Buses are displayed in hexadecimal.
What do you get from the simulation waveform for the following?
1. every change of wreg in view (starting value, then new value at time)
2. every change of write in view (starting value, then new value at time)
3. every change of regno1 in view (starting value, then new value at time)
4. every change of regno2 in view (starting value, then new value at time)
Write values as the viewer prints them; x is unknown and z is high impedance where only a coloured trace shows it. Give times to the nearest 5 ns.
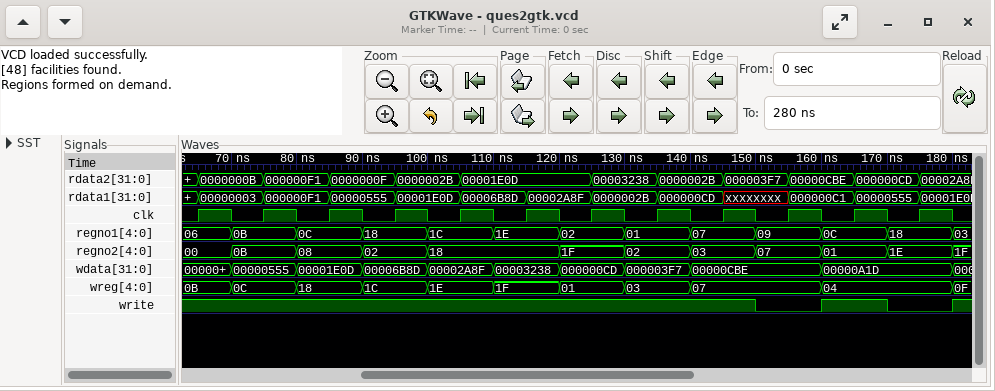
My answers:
0B, 0C at 70 ns, 18 at 80 ns, 1C at 90 ns, 1E at 100 ns, 1F at 110 ns, 01 at 120 ns, 03 at 130 ns, 07 at 140 ns, 04 at 160 ns, 0F at 180 ns
1, 0 at 150 ns, 1 at 160 ns, 0 at 170 ns, 1 at 180 ns
06, 0B at 70 ns, 0C at 80 ns, 18 at 90 ns, 1C at 100 ns, 1E at 110 ns, 02 at 120 ns, 01 at 130 ns, 07 at 140 ns, 09 at 150 ns, 0C at 160 ns, 18 at 170 ns, 03 at 180 ns
00, 0B at 70 ns, 08 at 80 ns, 02 at 90 ns, 18 at 100 ns, 1F at 120 ns, 02 at 130 ns, 03 at 140 ns, 07 at 150 ns, 01 at 160 ns, 1E at 170 ns, 1F at 180 ns
